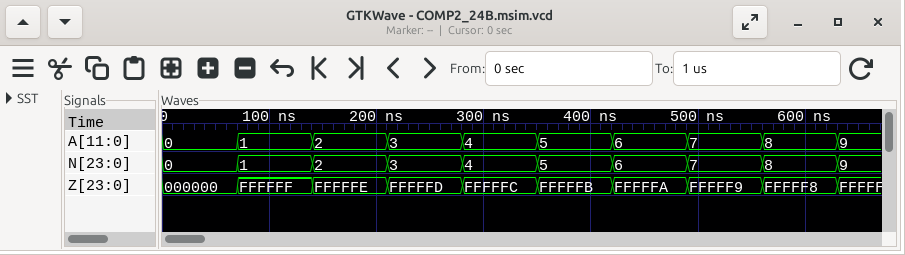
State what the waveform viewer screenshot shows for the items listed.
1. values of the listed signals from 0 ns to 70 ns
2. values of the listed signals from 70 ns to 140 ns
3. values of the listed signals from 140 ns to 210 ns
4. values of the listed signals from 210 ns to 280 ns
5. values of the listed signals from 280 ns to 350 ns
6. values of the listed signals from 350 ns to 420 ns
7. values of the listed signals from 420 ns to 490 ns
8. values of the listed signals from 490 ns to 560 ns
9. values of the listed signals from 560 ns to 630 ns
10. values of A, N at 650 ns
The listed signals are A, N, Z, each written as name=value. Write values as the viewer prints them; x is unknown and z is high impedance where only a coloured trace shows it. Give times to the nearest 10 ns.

A=0, N=0, Z=000000
A=1, N=1, Z=FFFFFF
A=2, N=2, Z=FFFFFE
A=3, N=3, Z=FFFFFD
A=4, N=4, Z=FFFFFC
A=5, N=5, Z=FFFFFB
A=6, N=6, Z=FFFFFA
A=7, N=7, Z=FFFFF9
A=8, N=8, Z=FFFFF8
A=9, N=9
